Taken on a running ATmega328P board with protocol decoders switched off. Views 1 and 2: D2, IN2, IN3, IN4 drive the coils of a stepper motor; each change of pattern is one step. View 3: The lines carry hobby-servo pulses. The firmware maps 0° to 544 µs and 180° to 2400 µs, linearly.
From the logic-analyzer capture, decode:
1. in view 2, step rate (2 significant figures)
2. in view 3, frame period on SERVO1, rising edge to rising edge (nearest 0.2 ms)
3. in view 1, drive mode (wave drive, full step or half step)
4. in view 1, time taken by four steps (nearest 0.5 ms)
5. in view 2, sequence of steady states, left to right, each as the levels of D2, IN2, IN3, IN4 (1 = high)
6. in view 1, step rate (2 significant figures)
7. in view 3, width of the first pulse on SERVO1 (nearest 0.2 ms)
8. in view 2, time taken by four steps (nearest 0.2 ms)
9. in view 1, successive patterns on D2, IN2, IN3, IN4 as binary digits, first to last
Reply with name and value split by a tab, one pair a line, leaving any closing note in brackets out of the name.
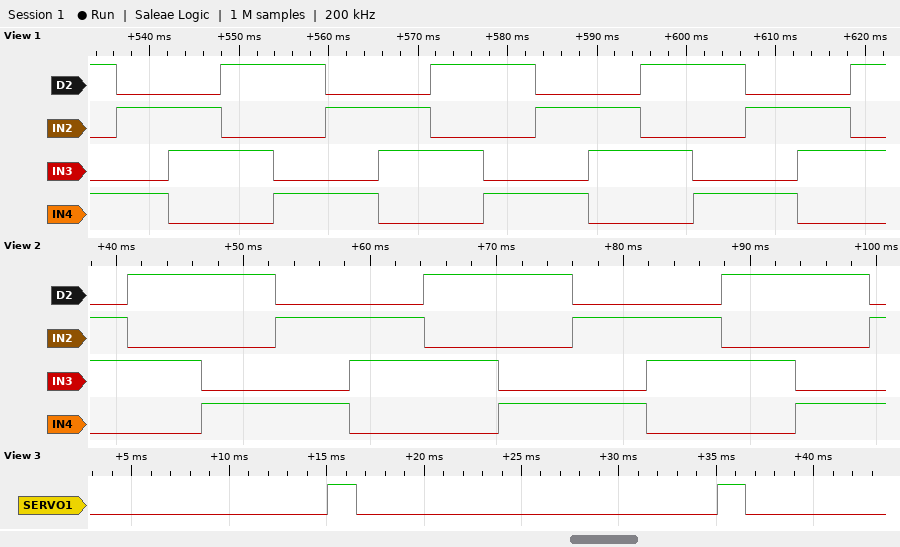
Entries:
in view 2, step rate	170 steps/s
in view 3, frame period on SERVO1, rising edge to rising edge	20.0 ms
in view 1, drive mode	full step
in view 1, time taken by four steps	23.5 ms
in view 2, sequence of steady states, left to right, each as the levels of D2, IN2, IN3, IN4	0110 1010 1001 0101 0110 1010 1001 0101 0110 1010 1001 0101
in view 1, step rate	170 steps/s
in view 3, width of the first pulse on SERVO1	1.4 ms
in view 2, time taken by four steps	23.4 ms
in view 1, successive patterns on D2, IN2, IN3, IN4 as binary digits, first to last	1001 0101 0110 1010 1001 0101 0110 1010 1001 0101 0110 1010 1001 0101 0110 1010
